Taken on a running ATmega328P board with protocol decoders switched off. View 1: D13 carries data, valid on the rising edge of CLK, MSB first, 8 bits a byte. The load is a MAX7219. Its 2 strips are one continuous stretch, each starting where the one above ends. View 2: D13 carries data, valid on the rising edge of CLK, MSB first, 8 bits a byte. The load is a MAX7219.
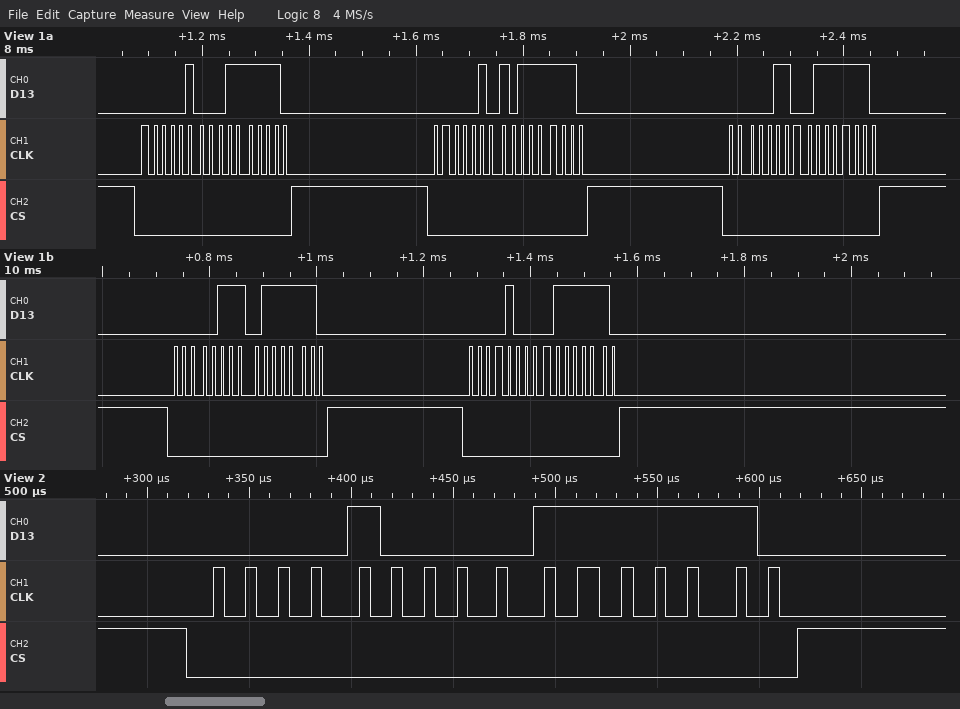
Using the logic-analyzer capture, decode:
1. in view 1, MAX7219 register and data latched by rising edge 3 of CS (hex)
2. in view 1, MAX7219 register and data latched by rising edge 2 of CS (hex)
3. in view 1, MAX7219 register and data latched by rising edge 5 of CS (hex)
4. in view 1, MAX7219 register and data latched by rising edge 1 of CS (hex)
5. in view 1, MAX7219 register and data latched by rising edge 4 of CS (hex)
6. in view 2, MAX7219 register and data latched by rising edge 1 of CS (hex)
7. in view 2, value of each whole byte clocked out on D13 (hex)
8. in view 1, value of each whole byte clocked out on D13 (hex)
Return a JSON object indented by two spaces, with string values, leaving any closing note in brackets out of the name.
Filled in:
{
  "in view 1, MAX7219 register and data latched by rising edge 3 of CS": "register 0x6, data 0x7E",
  "in view 1, MAX7219 register and data latched by rising edge 2 of CS": "register 0x5, data 0x7E",
  "in view 1, MAX7219 register and data latched by rising edge 5 of CS": "register 0x8, data 0x7E",
  "in view 1, MAX7219 register and data latched by rising edge 1 of CS": "register 0x4, data 0x7E",
  "in view 1, MAX7219 register and data latched by rising edge 4 of CS": "register 0x7, data 0x7E",
  "in view 2, MAX7219 register and data latched by rising edge 1 of CS": "register 0x8, data 0x7E",
  "in view 2, value of each whole byte clocked out on D13": "08 7E",
  "in view 1, value of each whole byte clocked out on D13": "04 7E 05 7E 06 7E 07 7E 08 7E"
}
